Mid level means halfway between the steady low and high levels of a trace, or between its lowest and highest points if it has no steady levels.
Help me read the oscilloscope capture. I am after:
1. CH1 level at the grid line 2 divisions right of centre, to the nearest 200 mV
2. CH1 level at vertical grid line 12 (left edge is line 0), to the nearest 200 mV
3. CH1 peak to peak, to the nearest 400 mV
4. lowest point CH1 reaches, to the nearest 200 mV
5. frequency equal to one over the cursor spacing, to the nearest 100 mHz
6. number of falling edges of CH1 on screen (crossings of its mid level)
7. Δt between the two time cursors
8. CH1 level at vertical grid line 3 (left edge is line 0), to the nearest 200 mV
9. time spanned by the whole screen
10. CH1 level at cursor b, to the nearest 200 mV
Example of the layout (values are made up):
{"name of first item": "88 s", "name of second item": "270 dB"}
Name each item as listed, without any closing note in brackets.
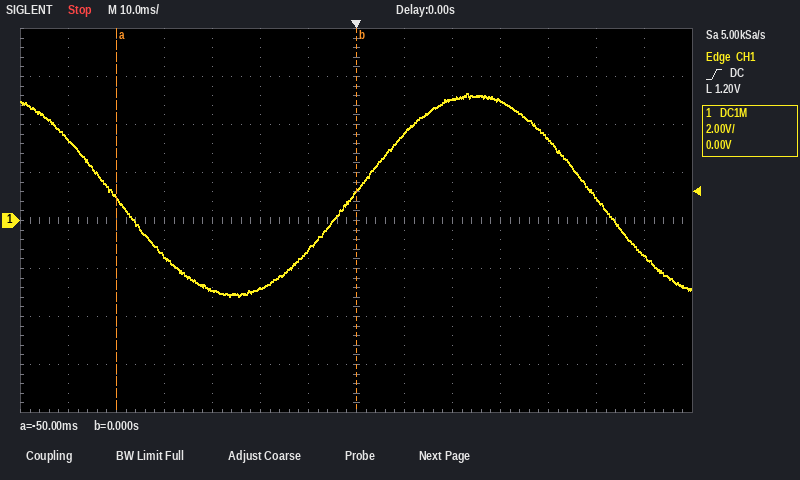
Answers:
{"CH1 level at the grid line 2 divisions right of centre, to the nearest 200 mV": "5.0 V", "CH1 level at vertical grid line 12 (left edge is line 0), to the nearest 200 mV": "1.0 V", "CH1 peak to peak, to the nearest 400 mV": "8.4 V", "lowest point CH1 reaches, to the nearest 200 mV": "-3.2 V", "frequency equal to one over the cursor spacing, to the nearest 100 mHz": "20.0 Hz", "number of falling edges of CH1 on screen": "2", "Δt between the two time cursors": "50 ms", "CH1 level at vertical grid line 3 (left edge is line 0), to the nearest 200 mV": "-1.4 V", "time spanned by the whole screen": "140 ms", "CH1 level at cursor b, to the nearest 200 mV": "1.2 V"}
